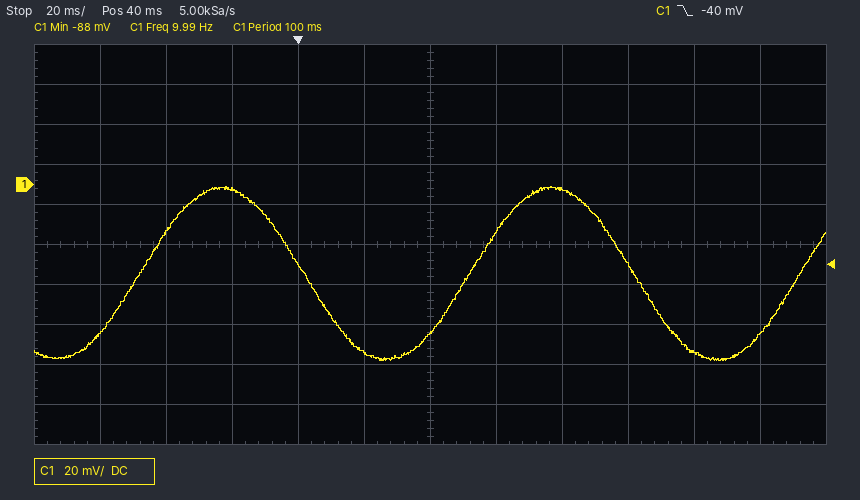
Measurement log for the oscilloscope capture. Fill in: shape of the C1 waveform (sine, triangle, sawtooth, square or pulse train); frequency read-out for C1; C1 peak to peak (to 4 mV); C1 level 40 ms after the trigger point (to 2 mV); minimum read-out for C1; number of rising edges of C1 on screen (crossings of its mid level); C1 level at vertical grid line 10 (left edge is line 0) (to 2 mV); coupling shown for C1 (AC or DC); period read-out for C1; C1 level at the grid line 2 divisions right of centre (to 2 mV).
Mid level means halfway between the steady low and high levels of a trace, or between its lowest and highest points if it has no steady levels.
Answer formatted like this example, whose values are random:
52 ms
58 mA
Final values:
sine
9.99 Hz
88 mV
-74 mV
-88 mV
3
-84 mV
DC
100 ms
-2 mV
